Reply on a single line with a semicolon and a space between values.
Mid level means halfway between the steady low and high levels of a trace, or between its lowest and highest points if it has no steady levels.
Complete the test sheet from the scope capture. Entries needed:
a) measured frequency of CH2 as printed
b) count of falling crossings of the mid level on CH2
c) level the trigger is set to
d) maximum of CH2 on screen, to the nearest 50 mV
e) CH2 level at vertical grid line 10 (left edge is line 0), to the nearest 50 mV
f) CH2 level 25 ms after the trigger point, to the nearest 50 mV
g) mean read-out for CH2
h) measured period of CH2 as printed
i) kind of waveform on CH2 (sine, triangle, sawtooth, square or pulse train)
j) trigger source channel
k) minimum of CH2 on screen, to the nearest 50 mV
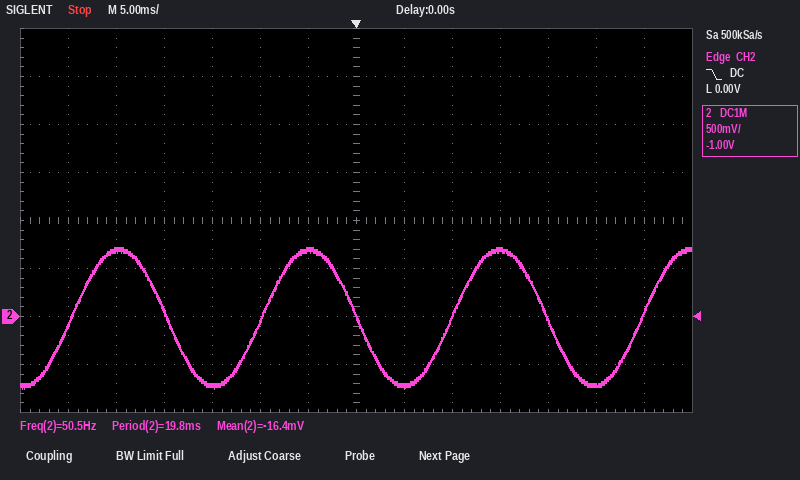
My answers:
50.5 Hz; 3; 0.00 V; 700 mV; 700 mV; -700 mV; -16.4 mV; 19.8 ms; sine; CH2; -750 mV
